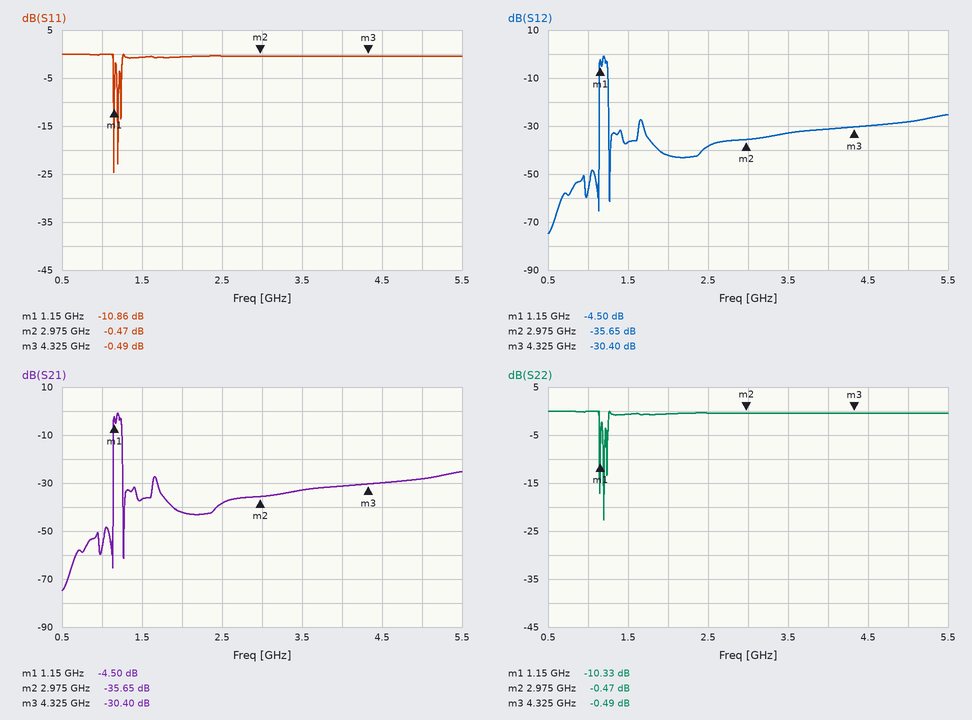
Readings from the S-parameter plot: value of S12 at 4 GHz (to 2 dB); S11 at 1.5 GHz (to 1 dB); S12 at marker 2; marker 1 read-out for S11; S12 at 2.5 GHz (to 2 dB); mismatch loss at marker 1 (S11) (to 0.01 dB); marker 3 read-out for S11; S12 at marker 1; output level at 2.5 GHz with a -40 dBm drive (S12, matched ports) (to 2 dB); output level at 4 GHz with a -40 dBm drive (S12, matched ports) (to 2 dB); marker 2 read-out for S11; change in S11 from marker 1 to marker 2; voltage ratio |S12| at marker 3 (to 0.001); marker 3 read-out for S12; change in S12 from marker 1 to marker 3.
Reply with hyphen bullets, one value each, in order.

- -32 dB
- -1 dB
- -35.65 dB
- -10.86 dB
- -38 dB
- 0.37 dB
- -0.49 dB
- -4.50 dB
- -78 dBm
- -72 dBm
- -0.47 dB
- 10.39 dB
- 0.030
- -30.40 dB
- -25.90 dB
